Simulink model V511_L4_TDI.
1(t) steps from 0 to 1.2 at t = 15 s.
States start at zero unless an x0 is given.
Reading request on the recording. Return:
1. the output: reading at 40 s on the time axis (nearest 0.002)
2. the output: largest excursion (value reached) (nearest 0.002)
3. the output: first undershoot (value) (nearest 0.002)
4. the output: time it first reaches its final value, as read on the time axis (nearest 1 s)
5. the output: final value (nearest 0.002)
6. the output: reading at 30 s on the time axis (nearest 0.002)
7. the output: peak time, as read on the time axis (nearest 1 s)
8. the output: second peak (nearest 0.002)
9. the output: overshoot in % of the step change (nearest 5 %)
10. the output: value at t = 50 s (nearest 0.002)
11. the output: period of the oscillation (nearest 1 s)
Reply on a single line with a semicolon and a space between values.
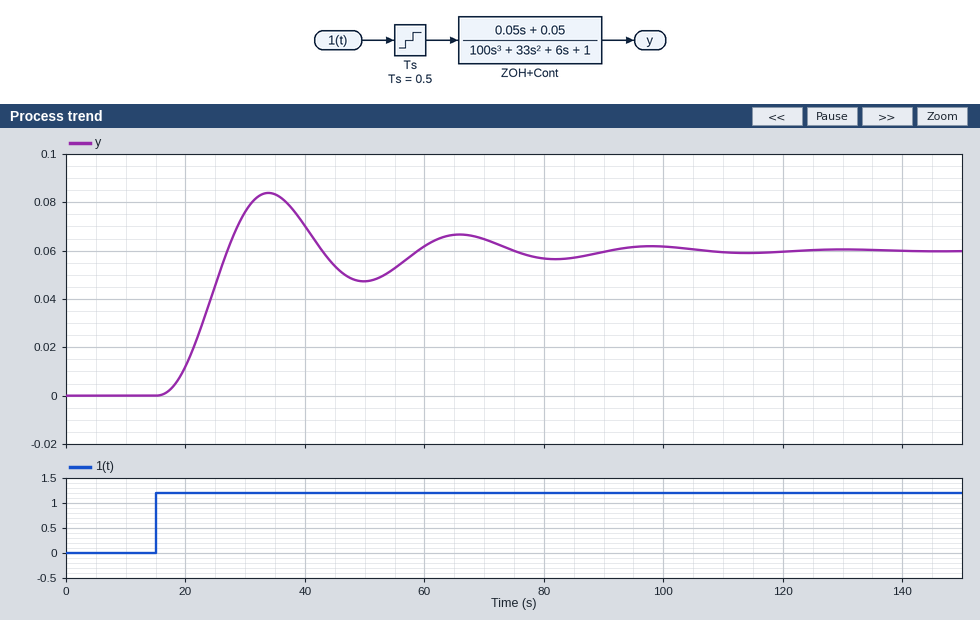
0.070; 0.084; 0.048; 27 s; 0.060; 0.076; 34 s; 0.066; 40 %; 0.048; 32 s
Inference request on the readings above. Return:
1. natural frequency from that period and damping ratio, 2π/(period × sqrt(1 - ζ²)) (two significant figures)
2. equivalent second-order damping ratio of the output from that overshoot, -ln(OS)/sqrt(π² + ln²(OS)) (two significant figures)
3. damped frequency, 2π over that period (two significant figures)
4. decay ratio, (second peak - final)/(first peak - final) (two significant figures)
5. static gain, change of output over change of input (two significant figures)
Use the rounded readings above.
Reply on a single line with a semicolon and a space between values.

0.20 rad/s; 0.28; 0.20 rad/s; 0.25; 0.050
